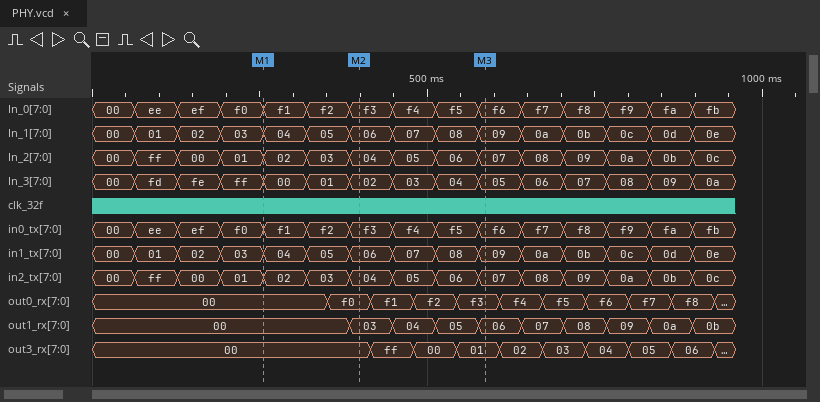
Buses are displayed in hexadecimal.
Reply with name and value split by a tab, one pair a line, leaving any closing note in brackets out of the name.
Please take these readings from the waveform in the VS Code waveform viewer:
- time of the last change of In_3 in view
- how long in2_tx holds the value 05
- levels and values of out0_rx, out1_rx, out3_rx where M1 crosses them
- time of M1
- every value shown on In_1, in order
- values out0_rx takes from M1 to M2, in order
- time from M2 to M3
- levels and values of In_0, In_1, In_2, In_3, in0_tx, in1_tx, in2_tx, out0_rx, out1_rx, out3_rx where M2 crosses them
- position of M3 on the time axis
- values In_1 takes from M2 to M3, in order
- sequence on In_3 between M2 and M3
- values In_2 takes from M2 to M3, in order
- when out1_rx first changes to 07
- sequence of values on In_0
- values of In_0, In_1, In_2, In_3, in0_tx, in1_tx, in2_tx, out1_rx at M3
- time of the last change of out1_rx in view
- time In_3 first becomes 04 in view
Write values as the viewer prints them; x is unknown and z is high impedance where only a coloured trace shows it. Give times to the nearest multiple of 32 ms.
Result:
time of the last change of In_3 in view	896 ms
how long in2_tx holds the value 05	64 ms
levels and values of out0_rx, out1_rx, out3_rx where M1 crosses them	out0_rx=00, out1_rx=00, out3_rx=00
time of M1	256 ms
every value shown on In_1, in order	00, 01, 02, 03, 04, 05, 06, 07, 08, 09, 0a, 0b, 0c, 0d, 0e
values out0_rx takes from M1 to M2, in order	00, f0
time from M2 to M3	192 ms
levels and values of In_0, In_1, In_2, In_3, in0_tx, in1_tx, in2_tx, out0_rx, out1_rx, out3_rx where M2 crosses them	In_0=f3, In_1=06, In_2=04, In_3=02, in0_tx=f3, in1_tx=06, in2_tx=04, out0_rx=f0, out1_rx=03, out3_rx=00
position of M3 on the time axis	576 ms
values In_1 takes from M2 to M3, in order	06, 07, 08, 09
sequence on In_3 between M2 and M3	02, 03, 04, 05
values In_2 takes from M2 to M3, in order	04, 05, 06, 07
when out1_rx first changes to 07	640 ms
sequence of values on In_0	00, ee, ef, f0, f1, f2, f3, f4, f5, f6, f7, f8, f9, fa, fb
values of In_0, In_1, In_2, In_3, in0_tx, in1_tx, in2_tx, out1_rx at M3	In_0=f6, In_1=09, In_2=07, In_3=05, in0_tx=f6, in1_tx=09, in2_tx=07, out1_rx=06
time of the last change of out1_rx in view	896 ms
time In_3 first becomes 04 in view	512 ms
